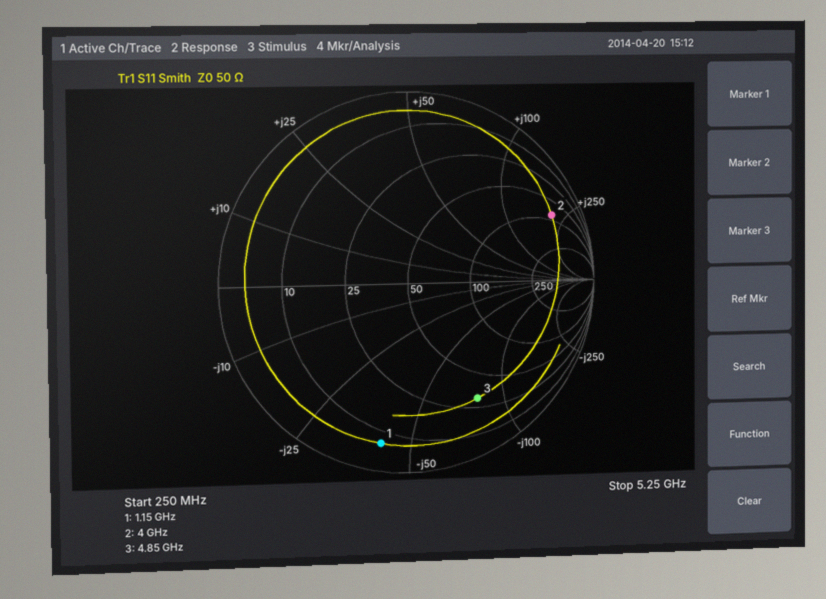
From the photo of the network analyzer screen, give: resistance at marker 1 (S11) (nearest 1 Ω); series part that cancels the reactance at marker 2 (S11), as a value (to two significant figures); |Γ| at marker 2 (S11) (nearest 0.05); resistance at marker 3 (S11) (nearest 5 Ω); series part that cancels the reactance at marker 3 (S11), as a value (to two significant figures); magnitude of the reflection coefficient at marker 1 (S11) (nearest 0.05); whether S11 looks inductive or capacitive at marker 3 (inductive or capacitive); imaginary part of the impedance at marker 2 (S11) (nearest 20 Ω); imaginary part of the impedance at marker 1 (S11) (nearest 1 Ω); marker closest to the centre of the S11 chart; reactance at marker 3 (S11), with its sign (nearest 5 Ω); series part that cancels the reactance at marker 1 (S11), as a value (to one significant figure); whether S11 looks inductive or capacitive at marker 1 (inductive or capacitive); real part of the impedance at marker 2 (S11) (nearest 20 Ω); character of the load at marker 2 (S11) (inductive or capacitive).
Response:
7 Ω
200 fF
0.85
30 Ω
2.6 nH
0.85
capacitive
+200 Ω
-41 Ω
marker 3
-80 Ω
6 nH
capacitive
80 Ω
inductive
